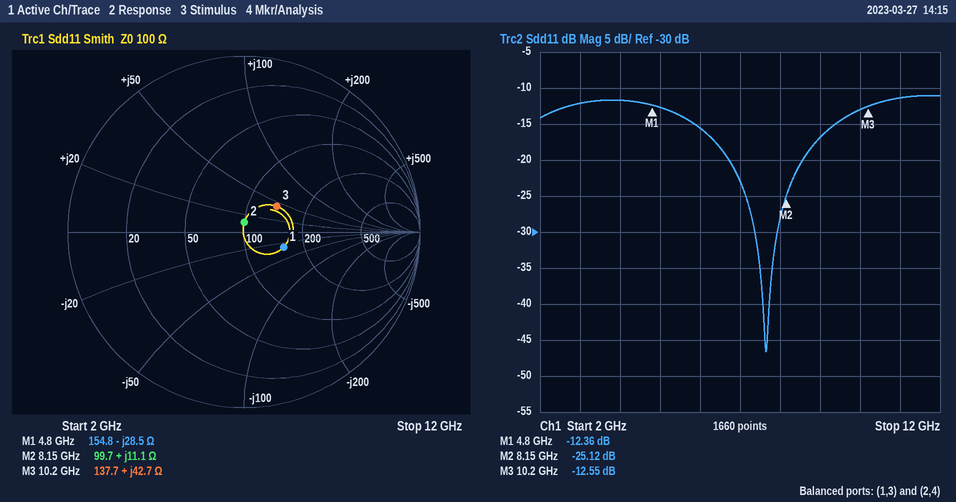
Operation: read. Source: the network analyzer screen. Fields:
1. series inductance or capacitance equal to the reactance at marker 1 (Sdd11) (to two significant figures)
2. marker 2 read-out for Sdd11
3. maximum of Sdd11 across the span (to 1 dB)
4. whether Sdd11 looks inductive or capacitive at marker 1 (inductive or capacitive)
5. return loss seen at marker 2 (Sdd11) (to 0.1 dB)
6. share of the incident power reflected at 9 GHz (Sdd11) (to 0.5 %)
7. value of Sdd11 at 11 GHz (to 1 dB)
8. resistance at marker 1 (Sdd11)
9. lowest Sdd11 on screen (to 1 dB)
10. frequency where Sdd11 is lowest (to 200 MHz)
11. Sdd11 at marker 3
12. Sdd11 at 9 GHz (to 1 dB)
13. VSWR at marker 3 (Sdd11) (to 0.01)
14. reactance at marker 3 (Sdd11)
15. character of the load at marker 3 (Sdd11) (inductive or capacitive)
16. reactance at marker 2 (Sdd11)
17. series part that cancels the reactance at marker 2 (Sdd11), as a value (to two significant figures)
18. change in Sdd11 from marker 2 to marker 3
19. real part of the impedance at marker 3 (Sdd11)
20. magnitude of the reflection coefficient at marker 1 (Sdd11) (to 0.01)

1.2 pF
-25.12 dB
-11 dB
capacitive
25.1 dB
2.0 %
-11 dB
154.8 Ω
-47 dB
7.6 GHz
-12.55 dB
-17 dB
1.62
+42.7 Ω
inductive
+11.1 Ω
1.8 pF
12.57 dB
137.7 Ω
0.24
